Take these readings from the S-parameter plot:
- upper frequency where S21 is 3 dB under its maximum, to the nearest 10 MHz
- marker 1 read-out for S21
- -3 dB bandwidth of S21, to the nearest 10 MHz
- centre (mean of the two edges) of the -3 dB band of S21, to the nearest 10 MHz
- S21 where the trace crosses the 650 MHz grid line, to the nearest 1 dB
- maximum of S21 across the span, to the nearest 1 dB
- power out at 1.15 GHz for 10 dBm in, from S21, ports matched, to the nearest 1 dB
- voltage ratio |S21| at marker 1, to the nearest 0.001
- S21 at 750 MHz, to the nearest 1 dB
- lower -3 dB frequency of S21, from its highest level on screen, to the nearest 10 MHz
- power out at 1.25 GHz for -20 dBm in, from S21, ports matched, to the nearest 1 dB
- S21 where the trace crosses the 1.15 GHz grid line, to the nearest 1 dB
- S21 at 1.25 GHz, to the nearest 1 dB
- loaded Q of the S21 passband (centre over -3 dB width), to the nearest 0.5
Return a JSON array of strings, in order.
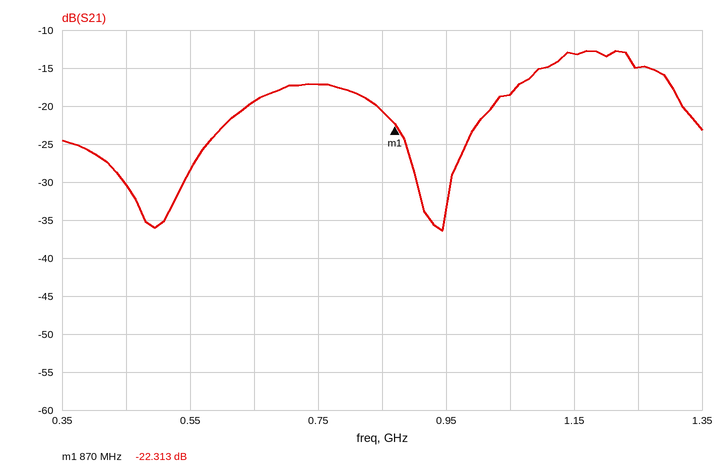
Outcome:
["1.29 GHz", "-22.313 dB", "200 MHz", "1.19 GHz", "-19 dB", "-13 dB", "-3 dBm", "0.077", "-17 dB", "1.09 GHz", "-35 dBm", "-13 dB", "-15 dB", "6.0"]
